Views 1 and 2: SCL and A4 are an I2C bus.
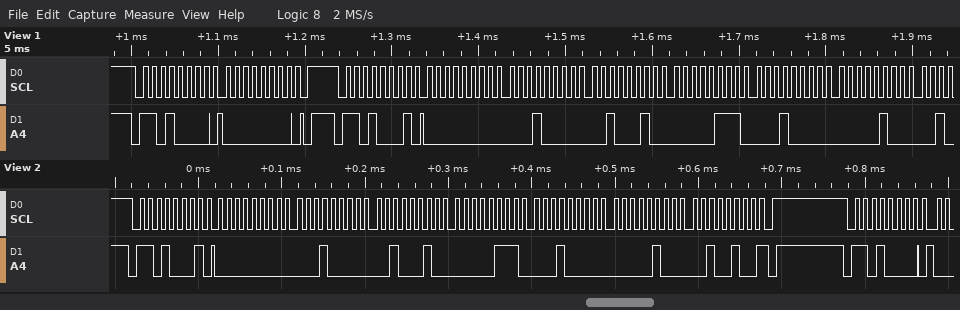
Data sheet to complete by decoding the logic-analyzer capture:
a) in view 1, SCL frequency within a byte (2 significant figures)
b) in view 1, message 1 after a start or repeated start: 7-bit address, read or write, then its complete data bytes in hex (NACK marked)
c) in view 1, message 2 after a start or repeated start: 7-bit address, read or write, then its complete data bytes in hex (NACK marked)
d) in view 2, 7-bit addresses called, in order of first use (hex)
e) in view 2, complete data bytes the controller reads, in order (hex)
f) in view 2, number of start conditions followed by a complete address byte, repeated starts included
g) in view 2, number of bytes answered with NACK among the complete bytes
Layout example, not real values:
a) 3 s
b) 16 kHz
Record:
a) 100 kHz
b) 0x68 write: 00
c) 0x68 read: 00 10 22 07 10 04
d) 0x68
e) 00 10 22 07 10 04 24
f) 2
g) 1
